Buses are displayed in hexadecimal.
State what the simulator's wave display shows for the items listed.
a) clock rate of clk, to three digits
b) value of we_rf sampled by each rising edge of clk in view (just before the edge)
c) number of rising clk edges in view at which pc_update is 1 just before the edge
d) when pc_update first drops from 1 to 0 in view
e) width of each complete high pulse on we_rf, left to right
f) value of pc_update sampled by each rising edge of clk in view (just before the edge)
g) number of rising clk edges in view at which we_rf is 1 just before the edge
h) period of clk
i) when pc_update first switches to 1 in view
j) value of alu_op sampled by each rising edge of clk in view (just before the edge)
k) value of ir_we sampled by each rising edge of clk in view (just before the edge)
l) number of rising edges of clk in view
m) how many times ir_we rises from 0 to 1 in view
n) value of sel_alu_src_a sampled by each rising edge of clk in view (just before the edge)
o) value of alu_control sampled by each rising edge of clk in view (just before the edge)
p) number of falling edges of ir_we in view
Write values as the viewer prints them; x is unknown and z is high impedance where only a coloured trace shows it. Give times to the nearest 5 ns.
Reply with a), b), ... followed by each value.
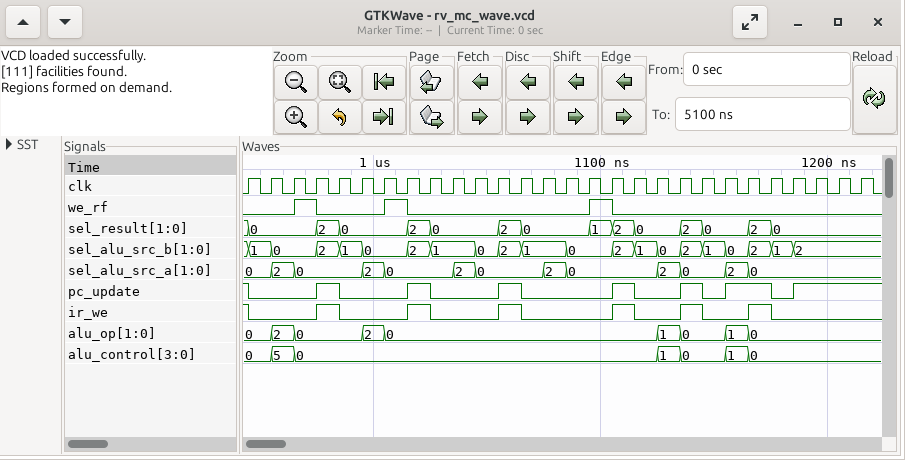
a) 100 MHz
b) 0 0 0 1 0 0 0 1 0 0 0 0 0 0 0 0 1 0 0 0 0 0 0 0 0 0 0 0
c) 11
d) 945 ns
e) 10 ns, 10 ns, 10 ns
f) 1 0 0 0 1 0 0 0 1 0 0 0 1 0 0 0 0 1 0 0 1 0 1 1 0 1 1 1
g) 3
h) 10 ns
i) 975 ns
j) 0, 0, 2, 0, 0, 0, 2, 0, 0, 0, 0, 0, 0, 0, 0, 0, 0, 0, 0, 1, 0, 0, 1, 0, 0, 0, 0, 0
k) 1 0 0 0 1 0 0 0 1 0 0 0 1 0 0 0 0 1 0 0 1 0 0 1 0 0 0 0
l) 28
m) 6
n) 0, 0, 2, 0, 0, 0, 2, 0, 0, 0, 2, 0, 0, 0, 2, 0, 0, 0, 0, 2, 0, 0, 2, 0, 0, 0, 0, 0
o) 0, 0, 5, 0, 0, 0, 0, 0, 0, 0, 0, 0, 0, 0, 0, 0, 0, 0, 0, 1, 0, 0, 1, 0, 0, 0, 0, 0
p) 7
